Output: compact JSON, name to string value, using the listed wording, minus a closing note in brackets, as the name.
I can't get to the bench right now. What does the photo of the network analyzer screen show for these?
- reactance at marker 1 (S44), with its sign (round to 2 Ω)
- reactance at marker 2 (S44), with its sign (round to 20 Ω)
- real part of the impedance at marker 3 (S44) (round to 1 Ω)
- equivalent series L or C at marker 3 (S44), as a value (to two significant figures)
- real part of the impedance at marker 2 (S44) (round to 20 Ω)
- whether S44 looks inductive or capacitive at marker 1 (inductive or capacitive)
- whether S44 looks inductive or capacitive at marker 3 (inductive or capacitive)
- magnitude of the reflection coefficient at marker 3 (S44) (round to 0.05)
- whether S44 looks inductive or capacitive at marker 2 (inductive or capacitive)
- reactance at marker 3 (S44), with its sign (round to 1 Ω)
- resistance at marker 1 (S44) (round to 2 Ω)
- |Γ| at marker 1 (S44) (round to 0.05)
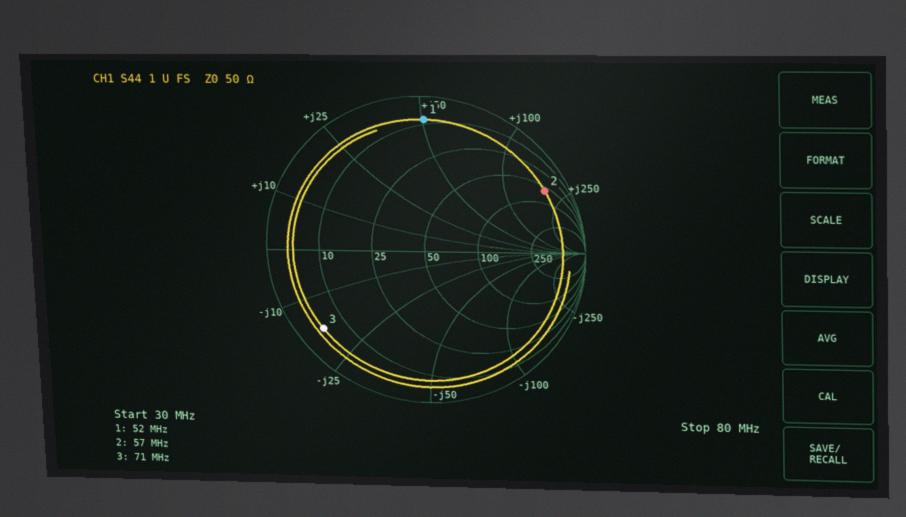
{"reactance at marker 1 (S44), with its sign": "+50 Ω", "reactance at marker 2 (S44), with its sign": "+180 Ω", "real part of the impedance at marker 3 (S44)": "5 Ω", "equivalent series L or C at marker 3 (S44), as a value": "130 pF", "real part of the impedance at marker 2 (S44)": "60 Ω", "whether S44 looks inductive or capacitive at marker 1": "inductive", "whether S44 looks inductive or capacitive at marker 3": "capacitive", "magnitude of the reflection coefficient at marker 3 (S44)": "0.85", "whether S44 looks inductive or capacitive at marker 2": "inductive", "reactance at marker 3 (S44), with its sign": "-17 Ω", "resistance at marker 1 (S44)": "8 Ω", "|Γ| at marker 1 (S44)": "0.85"}
